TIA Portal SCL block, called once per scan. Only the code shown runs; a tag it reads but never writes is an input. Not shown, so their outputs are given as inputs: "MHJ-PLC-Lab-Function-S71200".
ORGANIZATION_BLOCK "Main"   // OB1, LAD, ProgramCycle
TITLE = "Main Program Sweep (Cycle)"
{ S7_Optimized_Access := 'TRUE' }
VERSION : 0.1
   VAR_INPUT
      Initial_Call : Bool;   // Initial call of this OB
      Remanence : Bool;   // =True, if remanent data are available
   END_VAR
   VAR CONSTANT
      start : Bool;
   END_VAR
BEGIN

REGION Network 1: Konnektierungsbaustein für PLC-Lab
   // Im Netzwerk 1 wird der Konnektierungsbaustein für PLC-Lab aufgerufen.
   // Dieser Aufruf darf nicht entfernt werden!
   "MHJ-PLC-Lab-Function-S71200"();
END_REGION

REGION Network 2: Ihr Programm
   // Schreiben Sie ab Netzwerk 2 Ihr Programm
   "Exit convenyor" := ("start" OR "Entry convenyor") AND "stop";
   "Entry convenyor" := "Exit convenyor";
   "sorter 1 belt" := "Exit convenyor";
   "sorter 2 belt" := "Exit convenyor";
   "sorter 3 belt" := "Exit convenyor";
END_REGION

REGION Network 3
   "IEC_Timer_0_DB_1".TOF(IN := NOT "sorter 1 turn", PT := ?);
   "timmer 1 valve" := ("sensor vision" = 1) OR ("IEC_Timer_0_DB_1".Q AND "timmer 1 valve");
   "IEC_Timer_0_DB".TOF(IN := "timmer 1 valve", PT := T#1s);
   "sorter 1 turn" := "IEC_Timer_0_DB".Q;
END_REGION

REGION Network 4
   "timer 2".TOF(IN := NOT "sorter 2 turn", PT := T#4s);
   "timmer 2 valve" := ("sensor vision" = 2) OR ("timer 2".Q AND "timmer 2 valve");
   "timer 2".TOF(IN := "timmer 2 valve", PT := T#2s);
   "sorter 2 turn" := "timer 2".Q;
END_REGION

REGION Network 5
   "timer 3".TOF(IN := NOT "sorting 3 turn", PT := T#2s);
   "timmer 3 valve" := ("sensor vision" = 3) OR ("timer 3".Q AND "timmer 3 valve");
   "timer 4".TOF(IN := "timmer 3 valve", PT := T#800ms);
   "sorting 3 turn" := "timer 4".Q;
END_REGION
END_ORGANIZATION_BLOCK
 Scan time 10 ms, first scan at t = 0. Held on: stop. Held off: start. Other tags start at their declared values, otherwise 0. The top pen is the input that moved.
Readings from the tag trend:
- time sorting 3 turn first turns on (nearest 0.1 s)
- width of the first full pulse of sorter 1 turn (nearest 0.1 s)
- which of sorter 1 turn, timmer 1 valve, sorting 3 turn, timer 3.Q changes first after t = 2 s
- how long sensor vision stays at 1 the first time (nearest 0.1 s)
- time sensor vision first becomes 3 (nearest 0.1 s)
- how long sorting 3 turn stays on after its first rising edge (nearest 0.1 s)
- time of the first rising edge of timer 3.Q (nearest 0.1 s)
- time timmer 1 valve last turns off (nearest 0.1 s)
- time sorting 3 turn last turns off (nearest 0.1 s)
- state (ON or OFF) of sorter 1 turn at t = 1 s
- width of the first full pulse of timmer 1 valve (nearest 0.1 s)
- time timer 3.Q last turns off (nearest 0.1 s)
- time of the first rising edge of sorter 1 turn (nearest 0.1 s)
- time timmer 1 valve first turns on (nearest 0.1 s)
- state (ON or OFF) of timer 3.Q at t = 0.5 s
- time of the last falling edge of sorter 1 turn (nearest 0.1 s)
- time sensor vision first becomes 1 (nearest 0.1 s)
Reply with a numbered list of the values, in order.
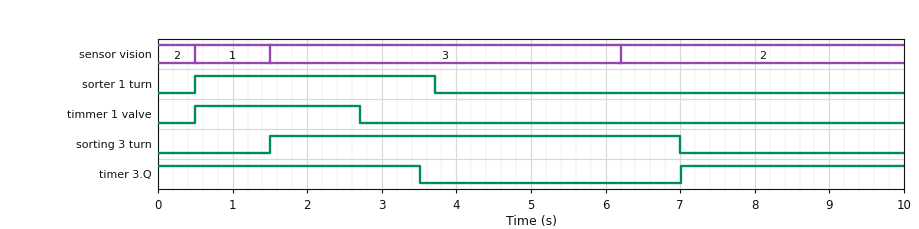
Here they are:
1. 1.5 s
2. 3.2 s
3. timmer 1 valve
4. 1.0 s
5. 1.5 s
6. 5.5 s
7. 7.0 s
8. 2.7 s
9. 7.0 s
10. ON
11. 2.2 s
12. 3.5 s
13. 0.5 s
14. 0.5 s
15. ON
16. 3.7 s
17. 0.5 s
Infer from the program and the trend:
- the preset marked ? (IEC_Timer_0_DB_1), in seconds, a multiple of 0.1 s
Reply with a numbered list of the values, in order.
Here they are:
1. 2.2 s
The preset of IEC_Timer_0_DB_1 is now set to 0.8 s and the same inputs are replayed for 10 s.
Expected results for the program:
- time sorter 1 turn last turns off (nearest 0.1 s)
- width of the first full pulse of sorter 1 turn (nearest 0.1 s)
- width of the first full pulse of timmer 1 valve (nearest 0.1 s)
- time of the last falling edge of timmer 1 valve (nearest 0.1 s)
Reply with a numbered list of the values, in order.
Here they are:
1. 2.5 s
2. 2.0 s
3. 1.0 s
4. 1.5 s
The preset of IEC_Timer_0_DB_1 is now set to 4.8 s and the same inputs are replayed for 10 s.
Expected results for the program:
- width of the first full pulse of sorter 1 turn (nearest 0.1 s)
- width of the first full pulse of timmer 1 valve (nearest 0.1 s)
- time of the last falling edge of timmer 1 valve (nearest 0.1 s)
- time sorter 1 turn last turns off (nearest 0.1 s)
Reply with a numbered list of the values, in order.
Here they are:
1. 5.8 s
2. 4.8 s
3. 5.3 s
4. 6.3 s
